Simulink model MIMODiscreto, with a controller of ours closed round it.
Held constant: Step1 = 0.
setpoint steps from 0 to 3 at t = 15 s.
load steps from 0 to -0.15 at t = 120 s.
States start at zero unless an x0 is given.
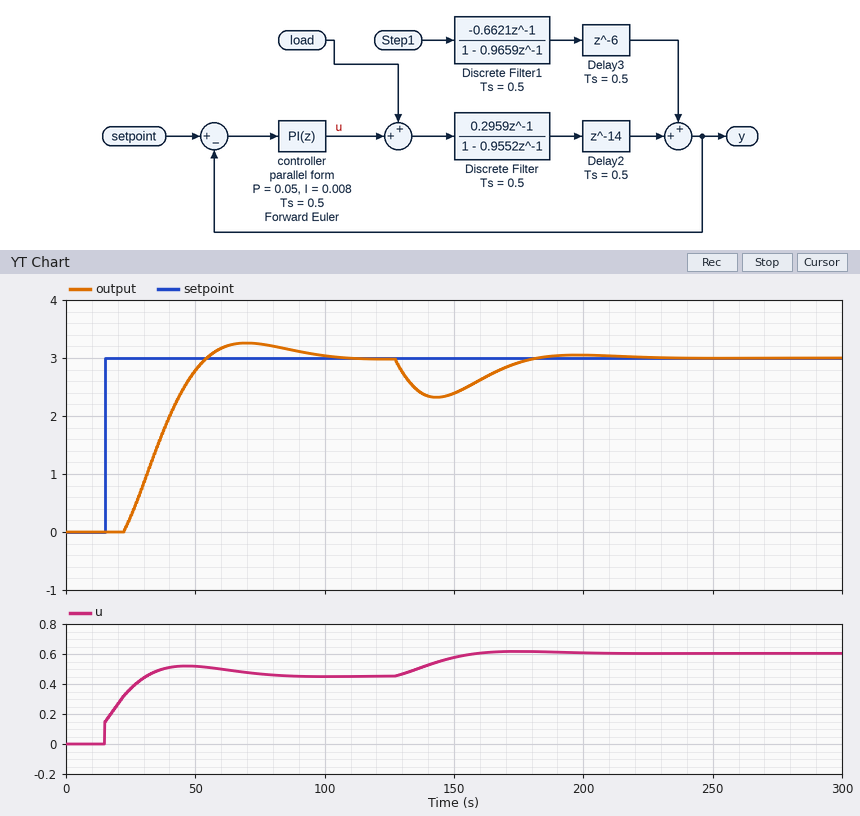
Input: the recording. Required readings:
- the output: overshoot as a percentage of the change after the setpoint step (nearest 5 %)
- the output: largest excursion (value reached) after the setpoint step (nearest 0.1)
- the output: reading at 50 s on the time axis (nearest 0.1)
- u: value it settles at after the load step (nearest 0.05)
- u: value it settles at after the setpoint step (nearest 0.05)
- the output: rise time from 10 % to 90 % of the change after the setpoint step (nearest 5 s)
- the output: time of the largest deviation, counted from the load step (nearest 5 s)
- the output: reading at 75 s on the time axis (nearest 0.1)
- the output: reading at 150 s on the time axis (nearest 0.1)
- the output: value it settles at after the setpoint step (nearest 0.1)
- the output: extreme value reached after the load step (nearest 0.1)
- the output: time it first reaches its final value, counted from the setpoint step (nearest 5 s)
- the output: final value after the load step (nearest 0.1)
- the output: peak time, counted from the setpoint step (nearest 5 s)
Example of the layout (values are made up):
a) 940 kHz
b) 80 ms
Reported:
a) 10 %
b) 3.3
c) 2.8
d) 0.60
e) 0.45
f) 25 s
g) 25 s
h) 3.2
i) 2.4
j) 3.0
k) 2.3
l) 40 s
m) 3.0
n) 55 s
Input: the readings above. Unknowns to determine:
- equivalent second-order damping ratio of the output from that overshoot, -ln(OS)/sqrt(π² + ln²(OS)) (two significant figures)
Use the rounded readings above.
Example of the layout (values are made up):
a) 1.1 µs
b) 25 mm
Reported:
a) 0.59
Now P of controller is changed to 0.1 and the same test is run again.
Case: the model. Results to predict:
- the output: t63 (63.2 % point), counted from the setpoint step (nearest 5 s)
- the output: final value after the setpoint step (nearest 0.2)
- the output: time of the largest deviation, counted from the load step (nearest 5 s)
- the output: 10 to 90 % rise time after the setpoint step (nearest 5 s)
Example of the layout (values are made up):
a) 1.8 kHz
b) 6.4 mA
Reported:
a) 20 s
b) 3.0
c) 20 s
d) 20 s
